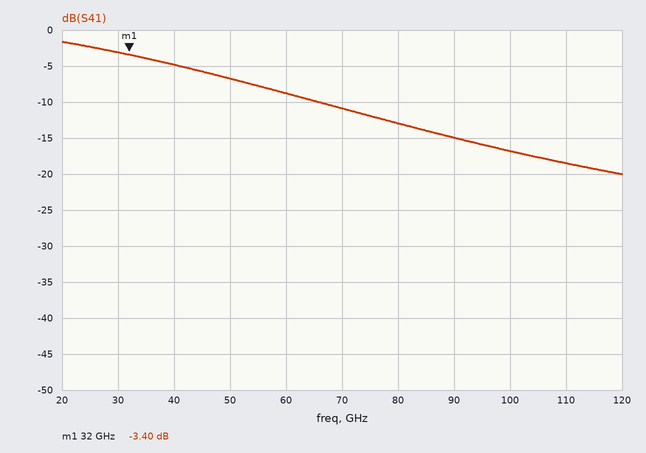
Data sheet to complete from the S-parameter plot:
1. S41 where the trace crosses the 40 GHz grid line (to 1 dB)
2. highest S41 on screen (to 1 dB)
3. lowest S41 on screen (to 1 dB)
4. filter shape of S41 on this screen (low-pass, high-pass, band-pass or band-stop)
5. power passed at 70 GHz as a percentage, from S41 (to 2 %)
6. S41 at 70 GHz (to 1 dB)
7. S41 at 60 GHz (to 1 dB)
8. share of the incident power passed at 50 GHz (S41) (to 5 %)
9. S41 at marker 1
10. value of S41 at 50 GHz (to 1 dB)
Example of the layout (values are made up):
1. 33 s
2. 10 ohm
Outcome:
1. -5 dB
2. -2 dB
3. -20 dB
4. low-pass
5. 8 %
6. -11 dB
7. -9 dB
8. 20 %
9. -3.40 dB
10. -7 dB
